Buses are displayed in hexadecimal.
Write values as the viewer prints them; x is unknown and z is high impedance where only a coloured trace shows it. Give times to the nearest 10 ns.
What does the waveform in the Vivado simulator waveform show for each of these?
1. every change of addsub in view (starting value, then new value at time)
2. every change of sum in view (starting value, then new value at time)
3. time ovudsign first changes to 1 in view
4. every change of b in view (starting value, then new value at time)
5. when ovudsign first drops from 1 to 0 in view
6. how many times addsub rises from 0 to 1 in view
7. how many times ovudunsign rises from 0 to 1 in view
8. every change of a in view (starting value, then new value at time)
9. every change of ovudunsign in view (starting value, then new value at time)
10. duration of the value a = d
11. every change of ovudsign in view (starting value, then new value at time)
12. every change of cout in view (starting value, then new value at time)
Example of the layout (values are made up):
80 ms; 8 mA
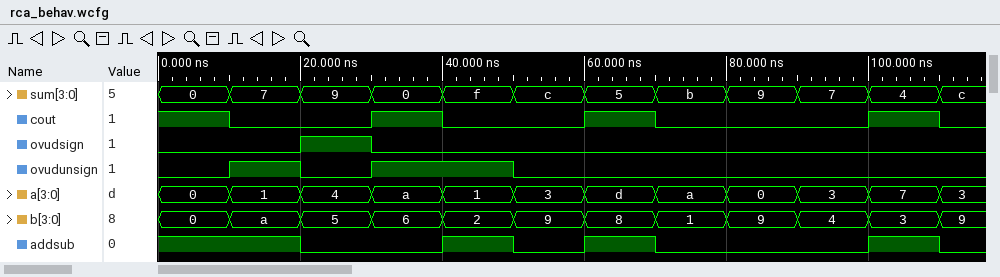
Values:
1, 0 at 20 ns, 1 at 40 ns, 0 at 50 ns, 1 at 60 ns, 0 at 70 ns, 1 at 100 ns, 0 at 110 ns; 0, 7 at 10 ns, 9 at 20 ns, 0 at 30 ns, f at 40 ns, c at 50 ns, 5 at 60 ns, b at 70 ns, 9 at 80 ns, 7 at 90 ns, 4 at 100 ns, c at 110 ns; 20 ns; 0, a at 10 ns, 5 at 20 ns, 6 at 30 ns, 2 at 40 ns, 9 at 50 ns, 8 at 60 ns, 1 at 70 ns, 9 at 80 ns, 4 at 90 ns, 3 at 100 ns, 9 at 110 ns; 30 ns; 3; 2; 0, 1 at 10 ns, 4 at 20 ns, a at 30 ns, 1 at 40 ns, 3 at 50 ns, d at 60 ns, a at 70 ns, 0 at 80 ns, 3 at 90 ns, 7 at 100 ns, 3 at 110 ns; 0, 1 at 10 ns, 0 at 20 ns, 1 at 30 ns, 0 at 50 ns; 10 ns; 0, 1 at 20 ns, 0 at 30 ns; 1, 0 at 10 ns, 1 at 30 ns, 0 at 40 ns, 1 at 60 ns, 0 at 70 ns, 1 at 100 ns, 0 at 110 ns
